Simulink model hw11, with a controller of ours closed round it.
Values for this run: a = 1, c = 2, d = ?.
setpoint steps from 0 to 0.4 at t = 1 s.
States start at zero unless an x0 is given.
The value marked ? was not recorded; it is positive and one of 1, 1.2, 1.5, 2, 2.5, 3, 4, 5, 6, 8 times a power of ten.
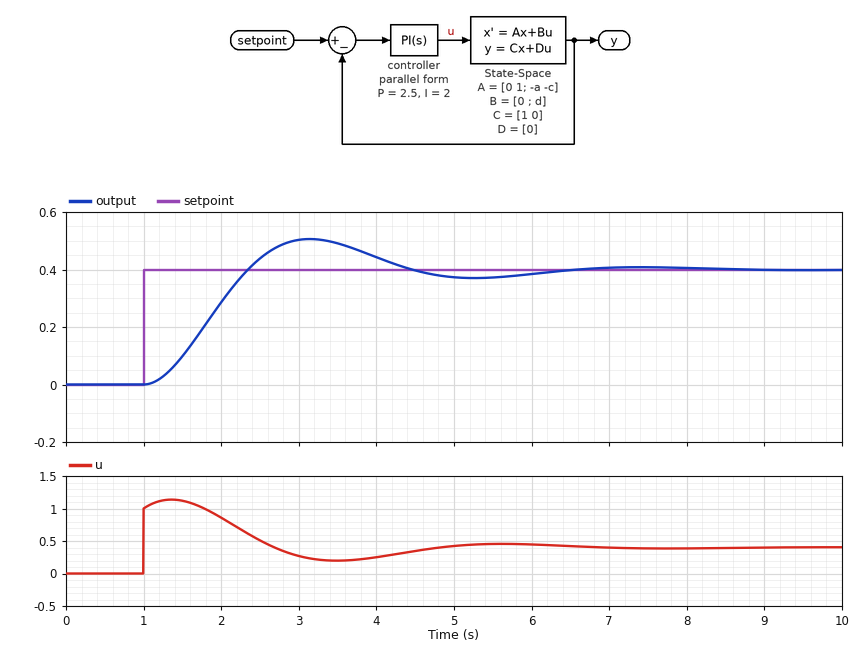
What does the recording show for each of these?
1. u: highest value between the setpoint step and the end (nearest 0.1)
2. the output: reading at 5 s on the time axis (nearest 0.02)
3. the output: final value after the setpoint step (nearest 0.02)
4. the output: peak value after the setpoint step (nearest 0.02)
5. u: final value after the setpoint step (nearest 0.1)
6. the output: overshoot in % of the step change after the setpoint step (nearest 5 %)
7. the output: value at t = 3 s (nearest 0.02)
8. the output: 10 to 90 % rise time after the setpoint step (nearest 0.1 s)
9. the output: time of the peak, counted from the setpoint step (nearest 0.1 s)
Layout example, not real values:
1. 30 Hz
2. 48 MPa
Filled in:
1. 1.1
2. 0.38
3. 0.40
4. 0.50
5. 0.4
6. 25 %
7. 0.50
8. 0.9 s
9. 2.1 s
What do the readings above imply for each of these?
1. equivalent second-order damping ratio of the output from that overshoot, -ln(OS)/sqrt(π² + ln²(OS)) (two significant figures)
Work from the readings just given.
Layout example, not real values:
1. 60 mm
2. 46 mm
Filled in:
1. 0.40
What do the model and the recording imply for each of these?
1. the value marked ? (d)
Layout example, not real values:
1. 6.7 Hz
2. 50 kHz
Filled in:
1. 1
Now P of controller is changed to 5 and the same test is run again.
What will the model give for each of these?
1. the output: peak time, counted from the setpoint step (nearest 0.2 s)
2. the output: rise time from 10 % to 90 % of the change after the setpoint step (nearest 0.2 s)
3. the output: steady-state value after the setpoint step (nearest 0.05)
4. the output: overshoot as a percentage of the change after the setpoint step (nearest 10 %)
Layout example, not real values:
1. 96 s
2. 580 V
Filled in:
1. 1.4 s
2. 0.6 s
3. 0.40
4. 20 %
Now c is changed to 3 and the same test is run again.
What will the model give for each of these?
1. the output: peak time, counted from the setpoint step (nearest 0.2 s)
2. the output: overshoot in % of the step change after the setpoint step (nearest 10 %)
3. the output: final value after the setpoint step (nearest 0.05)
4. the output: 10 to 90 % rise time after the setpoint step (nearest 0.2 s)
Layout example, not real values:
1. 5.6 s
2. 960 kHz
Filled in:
1. 2.8 s
2. 20 %
3. 0.40
4. 1.2 s
